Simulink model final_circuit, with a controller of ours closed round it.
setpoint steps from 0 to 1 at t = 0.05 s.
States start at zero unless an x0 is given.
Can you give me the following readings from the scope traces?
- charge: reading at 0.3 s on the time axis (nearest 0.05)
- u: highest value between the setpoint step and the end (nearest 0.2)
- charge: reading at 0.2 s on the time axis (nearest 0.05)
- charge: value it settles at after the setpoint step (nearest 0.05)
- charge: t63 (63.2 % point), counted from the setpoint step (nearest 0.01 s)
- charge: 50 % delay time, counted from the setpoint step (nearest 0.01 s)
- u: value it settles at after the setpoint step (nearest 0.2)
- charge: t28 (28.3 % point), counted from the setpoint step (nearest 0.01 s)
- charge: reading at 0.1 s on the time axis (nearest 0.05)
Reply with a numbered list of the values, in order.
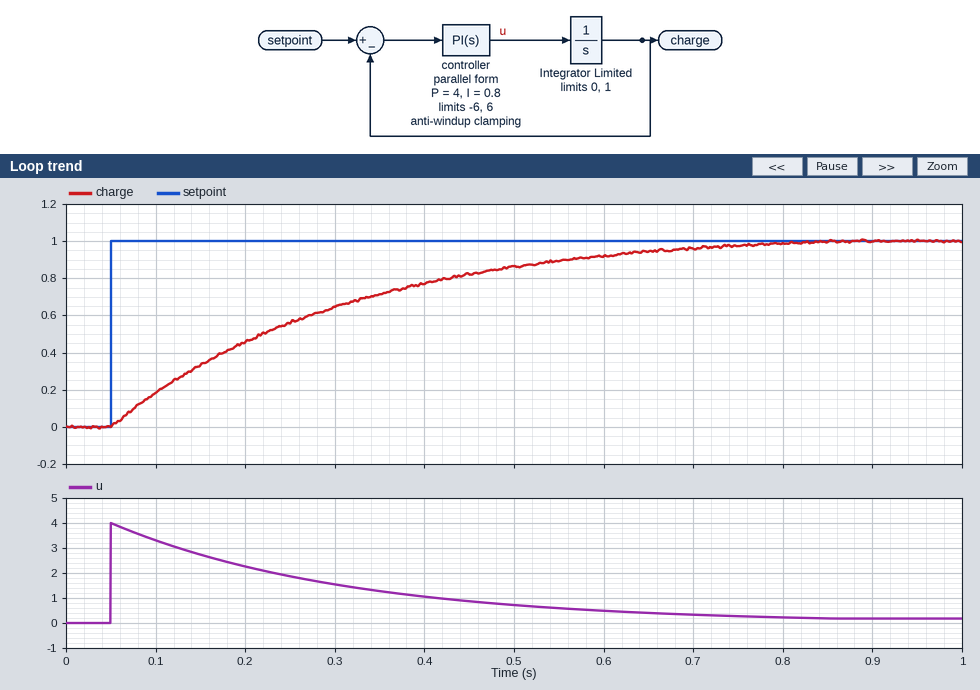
1. 0.65
2. 4.0
3. 0.45
4. 1.00
5. 0.24 s
6. 0.17 s
7. 0.2
8. 0.08 s
9. 0.20
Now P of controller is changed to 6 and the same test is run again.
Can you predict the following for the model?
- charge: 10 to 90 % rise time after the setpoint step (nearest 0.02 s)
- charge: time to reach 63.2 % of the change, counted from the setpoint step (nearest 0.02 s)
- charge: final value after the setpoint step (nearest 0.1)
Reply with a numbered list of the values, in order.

1. 0.34 s
2. 0.16 s
3. 1.0
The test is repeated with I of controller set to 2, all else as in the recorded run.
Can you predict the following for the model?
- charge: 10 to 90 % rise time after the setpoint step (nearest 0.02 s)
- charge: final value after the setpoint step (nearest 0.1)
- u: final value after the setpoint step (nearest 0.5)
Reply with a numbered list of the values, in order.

1. 0.42 s
2. 1.0
3. 0.5
